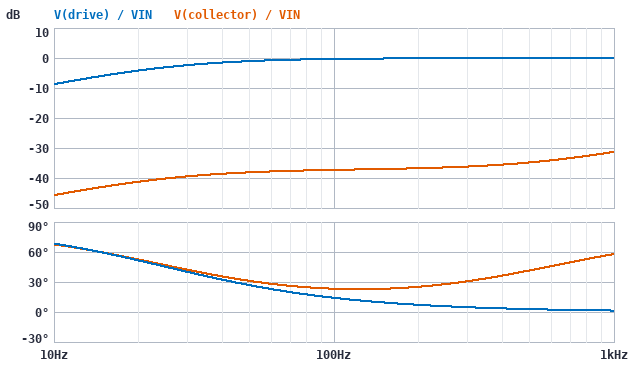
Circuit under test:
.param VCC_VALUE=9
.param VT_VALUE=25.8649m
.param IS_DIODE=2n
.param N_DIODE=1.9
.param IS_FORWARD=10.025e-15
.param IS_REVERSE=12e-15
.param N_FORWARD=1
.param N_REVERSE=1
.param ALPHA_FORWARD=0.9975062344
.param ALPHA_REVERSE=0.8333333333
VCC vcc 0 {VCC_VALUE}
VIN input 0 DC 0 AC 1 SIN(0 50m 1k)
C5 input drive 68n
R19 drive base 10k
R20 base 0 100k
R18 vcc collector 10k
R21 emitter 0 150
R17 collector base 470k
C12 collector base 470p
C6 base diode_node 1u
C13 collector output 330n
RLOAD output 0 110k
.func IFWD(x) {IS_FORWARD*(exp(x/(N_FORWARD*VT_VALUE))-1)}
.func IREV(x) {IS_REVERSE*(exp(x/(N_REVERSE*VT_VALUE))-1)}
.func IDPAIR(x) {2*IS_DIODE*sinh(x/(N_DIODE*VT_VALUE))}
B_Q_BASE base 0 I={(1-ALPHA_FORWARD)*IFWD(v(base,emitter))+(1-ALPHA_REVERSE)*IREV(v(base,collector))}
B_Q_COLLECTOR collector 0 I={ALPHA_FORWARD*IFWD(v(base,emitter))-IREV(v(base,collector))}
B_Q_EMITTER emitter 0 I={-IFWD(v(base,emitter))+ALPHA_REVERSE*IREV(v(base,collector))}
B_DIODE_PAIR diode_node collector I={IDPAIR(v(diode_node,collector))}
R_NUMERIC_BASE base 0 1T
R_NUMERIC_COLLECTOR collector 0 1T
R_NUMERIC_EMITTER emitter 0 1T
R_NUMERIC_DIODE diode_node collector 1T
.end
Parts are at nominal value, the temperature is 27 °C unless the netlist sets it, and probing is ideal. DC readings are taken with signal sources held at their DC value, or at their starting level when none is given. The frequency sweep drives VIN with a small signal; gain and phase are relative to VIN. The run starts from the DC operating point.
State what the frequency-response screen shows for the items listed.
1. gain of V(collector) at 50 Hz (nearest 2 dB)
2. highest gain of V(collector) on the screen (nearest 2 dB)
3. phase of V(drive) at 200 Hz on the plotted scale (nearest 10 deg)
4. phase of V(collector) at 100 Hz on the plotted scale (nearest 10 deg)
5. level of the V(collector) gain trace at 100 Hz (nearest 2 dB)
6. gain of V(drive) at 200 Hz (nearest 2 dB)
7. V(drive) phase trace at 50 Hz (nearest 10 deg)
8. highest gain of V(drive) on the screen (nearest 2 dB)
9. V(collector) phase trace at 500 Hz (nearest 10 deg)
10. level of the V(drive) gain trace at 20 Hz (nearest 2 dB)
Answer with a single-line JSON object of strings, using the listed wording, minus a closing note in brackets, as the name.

{"gain of V(collector) at 50 Hz": "-38 dB", "highest gain of V(collector) on the screen": "-32 dB", "phase of V(drive) at 200 Hz on the plotted scale": "10 deg", "phase of V(collector) at 100 Hz on the plotted scale": "20 deg", "level of the V(collector) gain trace at 100 Hz": "-38 dB", "gain of V(drive) at 200 Hz": "0 dB", "V(drive) phase trace at 50 Hz": "30 deg", "highest gain of V(drive) on the screen": "0 dB", "V(collector) phase trace at 500 Hz": "40 deg", "level of the V(drive) gain trace at 20 Hz": "-4 dB"}
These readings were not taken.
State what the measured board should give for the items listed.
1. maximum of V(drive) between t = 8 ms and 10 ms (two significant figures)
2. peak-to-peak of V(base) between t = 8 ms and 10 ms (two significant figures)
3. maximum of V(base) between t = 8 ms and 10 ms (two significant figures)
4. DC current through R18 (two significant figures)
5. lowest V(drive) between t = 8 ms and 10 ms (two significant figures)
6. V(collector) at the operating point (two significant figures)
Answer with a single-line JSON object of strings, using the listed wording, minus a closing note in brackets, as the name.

{"maximum of V(drive) between t = 8 ms and 10 ms": "1.6 V", "peak-to-peak of V(base) between t = 8 ms and 10 ms": "89 mV", "maximum of V(base) between t = 8 ms and 10 ms": "1.6 V", "DC current through R18": "16 µA", "lowest V(drive) between t = 8 ms and 10 ms": "1.5 V", "V(collector) at the operating point": "8.8 V"}
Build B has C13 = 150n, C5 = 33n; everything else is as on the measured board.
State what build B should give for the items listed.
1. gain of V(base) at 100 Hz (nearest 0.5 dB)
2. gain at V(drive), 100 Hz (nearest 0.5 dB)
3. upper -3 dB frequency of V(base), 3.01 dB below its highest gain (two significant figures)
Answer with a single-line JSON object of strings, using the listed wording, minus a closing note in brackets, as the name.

{"gain of V(base) at 100 Hz": "-2.0 dB", "gain at V(drive), 100 Hz": "-1.0 dB", "upper -3 dB frequency of V(base), 3.01 dB below its highest gain": "29 kHz"}
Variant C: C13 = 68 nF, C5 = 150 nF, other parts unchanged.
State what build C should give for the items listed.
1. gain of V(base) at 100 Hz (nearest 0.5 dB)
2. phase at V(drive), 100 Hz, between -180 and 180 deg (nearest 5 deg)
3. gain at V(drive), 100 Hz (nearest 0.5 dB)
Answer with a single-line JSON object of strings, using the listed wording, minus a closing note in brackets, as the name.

{"gain of V(base) at 100 Hz": "-1.0 dB", "phase at V(drive), 100 Hz, between -180 and 180 deg": "5 deg", "gain at V(drive), 100 Hz": "0 dB"}
